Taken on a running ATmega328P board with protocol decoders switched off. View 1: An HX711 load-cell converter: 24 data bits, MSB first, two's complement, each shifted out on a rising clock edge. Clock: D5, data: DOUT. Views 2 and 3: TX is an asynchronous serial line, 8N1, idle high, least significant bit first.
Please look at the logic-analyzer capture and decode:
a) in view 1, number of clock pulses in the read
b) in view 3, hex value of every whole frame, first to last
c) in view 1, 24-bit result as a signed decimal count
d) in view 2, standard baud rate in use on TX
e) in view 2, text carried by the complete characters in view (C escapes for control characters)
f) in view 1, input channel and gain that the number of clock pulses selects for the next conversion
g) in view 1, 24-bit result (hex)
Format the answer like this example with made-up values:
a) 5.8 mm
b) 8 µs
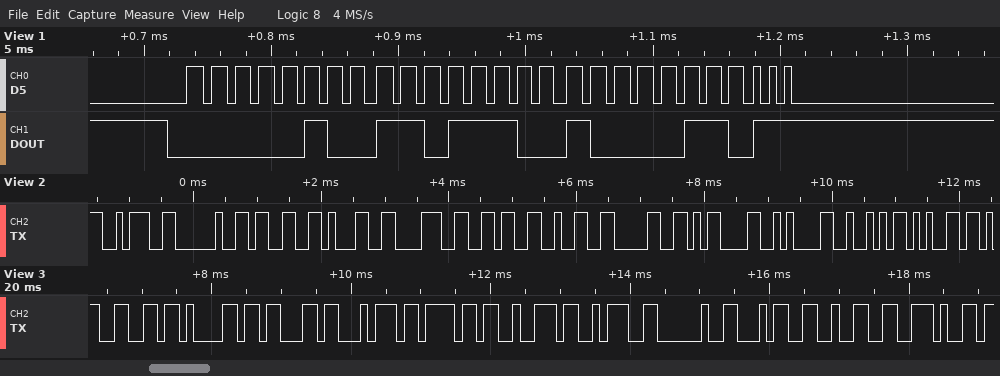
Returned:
a) 27
b) 0x66 0x61 0x63 0x74 0x6F 0x72 0x3A 0x20 0x34 0x32 0x2E
c) 318598
d) 9600 baud
e) ": 318620\r\nRe"
f) channel A, gain 64
g) 0x04DC86
